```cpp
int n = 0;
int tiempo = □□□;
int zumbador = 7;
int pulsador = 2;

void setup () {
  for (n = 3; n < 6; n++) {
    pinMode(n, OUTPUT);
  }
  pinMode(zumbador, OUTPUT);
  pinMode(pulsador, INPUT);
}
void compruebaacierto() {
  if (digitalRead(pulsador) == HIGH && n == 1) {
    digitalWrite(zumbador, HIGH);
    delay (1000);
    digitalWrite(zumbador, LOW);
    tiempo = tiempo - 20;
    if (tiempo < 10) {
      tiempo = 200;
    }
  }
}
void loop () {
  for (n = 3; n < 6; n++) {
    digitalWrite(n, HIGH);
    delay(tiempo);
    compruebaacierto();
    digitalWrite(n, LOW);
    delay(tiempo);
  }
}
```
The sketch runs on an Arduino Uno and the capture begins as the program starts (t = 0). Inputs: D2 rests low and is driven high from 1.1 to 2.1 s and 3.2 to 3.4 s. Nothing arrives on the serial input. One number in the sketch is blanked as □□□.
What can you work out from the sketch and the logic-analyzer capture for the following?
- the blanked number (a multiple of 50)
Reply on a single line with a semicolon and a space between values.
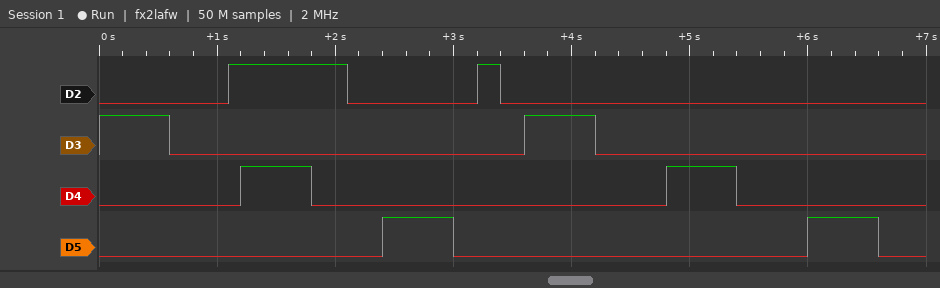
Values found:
600
